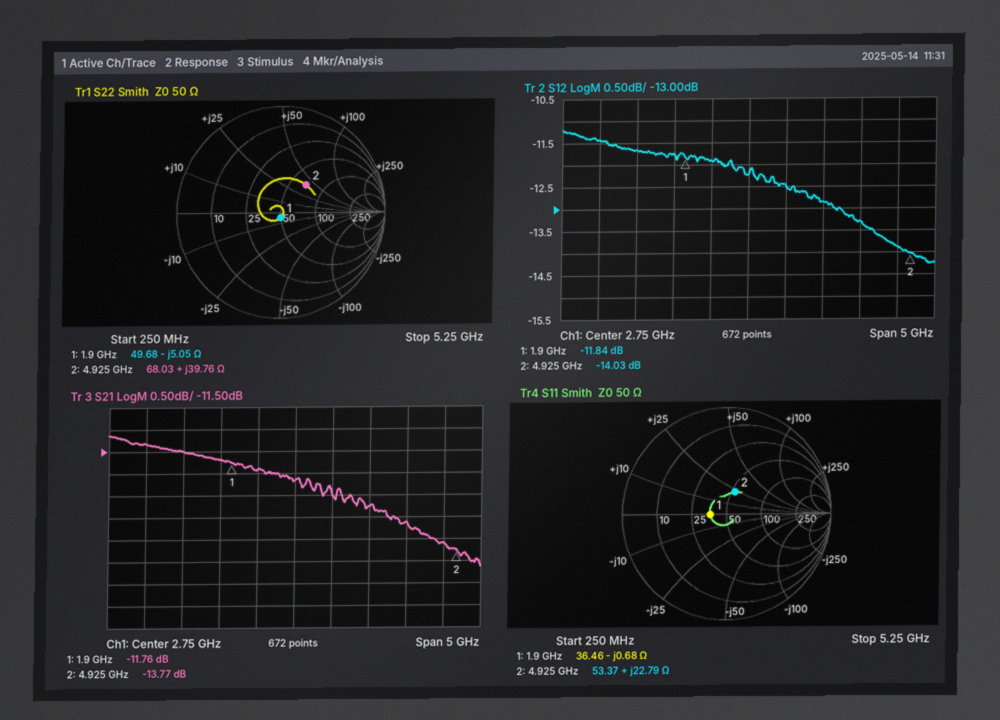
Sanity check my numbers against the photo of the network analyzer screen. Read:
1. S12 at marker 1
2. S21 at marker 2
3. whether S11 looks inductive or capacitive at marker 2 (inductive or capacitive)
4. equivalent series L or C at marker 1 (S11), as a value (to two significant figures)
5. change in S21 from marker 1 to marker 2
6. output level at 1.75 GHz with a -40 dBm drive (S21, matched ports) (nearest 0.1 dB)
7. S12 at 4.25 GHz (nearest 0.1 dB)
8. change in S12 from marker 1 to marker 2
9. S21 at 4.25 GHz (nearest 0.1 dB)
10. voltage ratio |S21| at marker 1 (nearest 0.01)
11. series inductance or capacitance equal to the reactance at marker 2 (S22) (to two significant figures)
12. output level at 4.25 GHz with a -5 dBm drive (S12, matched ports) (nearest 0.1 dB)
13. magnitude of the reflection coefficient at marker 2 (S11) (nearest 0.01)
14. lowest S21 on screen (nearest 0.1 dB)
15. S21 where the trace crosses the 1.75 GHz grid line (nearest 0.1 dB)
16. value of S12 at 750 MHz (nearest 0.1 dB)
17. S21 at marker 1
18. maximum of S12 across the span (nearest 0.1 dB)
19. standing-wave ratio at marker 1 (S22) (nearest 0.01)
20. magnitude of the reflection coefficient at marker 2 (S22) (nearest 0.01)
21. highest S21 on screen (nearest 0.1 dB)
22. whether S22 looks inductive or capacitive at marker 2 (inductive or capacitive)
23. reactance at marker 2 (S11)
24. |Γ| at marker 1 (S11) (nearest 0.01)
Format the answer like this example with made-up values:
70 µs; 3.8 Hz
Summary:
-11.84 dB; -13.77 dB; inductive; 120 pF; -2.01 dB; -51.7 dBm; -13.3 dB; -2.19 dB; -13.1 dB; 0.26; 1.3 nH; -18.3 dBm; 0.22; -14.1 dB; -11.7 dB; -11.4 dB; -11.76 dB; -11.2 dB; 1.11; 0.35; -11.1 dB; inductive; +22.79 Ω; 0.16
